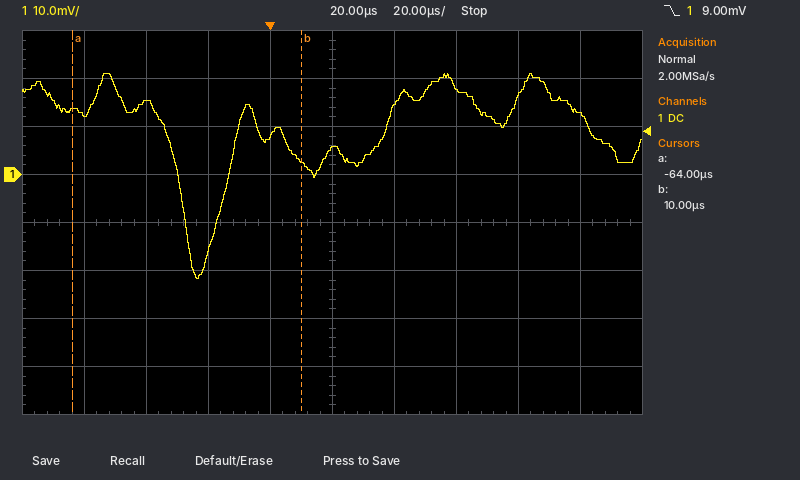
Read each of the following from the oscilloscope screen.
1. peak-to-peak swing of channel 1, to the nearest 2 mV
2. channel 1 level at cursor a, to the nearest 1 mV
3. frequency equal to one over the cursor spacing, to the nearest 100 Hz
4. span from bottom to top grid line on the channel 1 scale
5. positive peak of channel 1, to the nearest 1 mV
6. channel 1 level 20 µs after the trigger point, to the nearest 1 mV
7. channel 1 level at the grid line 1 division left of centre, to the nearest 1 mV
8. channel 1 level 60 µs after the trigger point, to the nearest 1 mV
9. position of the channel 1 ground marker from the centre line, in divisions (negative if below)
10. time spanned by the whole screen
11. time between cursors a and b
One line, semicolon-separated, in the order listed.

42 mV; 13 mV; 13.5 kHz; 80 mV; 21 mV; 5 mV; 8 mV; 18 mV; +1.0 div; 200 µs; 74 µs
